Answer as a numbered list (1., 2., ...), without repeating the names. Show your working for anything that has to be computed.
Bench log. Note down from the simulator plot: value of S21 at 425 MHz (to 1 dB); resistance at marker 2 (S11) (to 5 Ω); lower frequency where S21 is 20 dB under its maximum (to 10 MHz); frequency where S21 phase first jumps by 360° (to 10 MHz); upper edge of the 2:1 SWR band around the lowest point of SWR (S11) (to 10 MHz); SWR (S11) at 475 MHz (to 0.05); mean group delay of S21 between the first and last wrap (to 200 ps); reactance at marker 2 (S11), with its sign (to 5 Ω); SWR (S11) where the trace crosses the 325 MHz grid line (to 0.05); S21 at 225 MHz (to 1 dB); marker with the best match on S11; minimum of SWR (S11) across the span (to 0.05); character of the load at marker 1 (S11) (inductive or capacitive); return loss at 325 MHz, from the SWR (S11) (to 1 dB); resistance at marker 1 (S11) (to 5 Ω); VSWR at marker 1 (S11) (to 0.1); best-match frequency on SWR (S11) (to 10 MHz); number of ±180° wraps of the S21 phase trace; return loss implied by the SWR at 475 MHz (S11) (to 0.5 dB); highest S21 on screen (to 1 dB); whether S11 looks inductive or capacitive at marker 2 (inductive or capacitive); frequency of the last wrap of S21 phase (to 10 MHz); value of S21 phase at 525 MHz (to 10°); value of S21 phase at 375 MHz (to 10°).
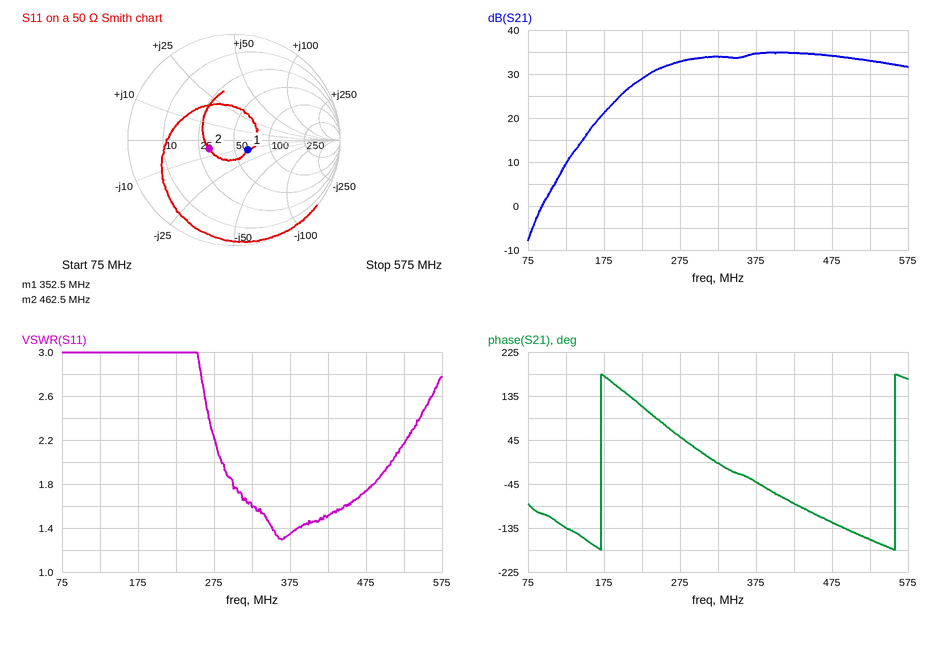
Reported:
1. 35 dB
2. 30 Ω
3. 150 MHz
4. 170 MHz
5. 510 MHz
6. 1.75
7. 1 cycle / (560 MHz − 170 MHz) ≈ 2.6 ns
8. -5 Ω
9. 1.60
10. 29 dB
11. marker 1
12. 1.30
13. capacitive
14. −20 log10((1.6 − 1)/(1.6 + 1)) ≈ 13 dB
15. 65 Ω
16. 1.4
17. 360 MHz
18. 2
19. −20 log10((1.75 − 1)/(1.75 + 1)) ≈ 11.3 dB, so 11.5 dB to the nearest 0.5 dB
20. 35 dB
21. capacitive
22. 560 MHz
23. -160°
24. -40°
